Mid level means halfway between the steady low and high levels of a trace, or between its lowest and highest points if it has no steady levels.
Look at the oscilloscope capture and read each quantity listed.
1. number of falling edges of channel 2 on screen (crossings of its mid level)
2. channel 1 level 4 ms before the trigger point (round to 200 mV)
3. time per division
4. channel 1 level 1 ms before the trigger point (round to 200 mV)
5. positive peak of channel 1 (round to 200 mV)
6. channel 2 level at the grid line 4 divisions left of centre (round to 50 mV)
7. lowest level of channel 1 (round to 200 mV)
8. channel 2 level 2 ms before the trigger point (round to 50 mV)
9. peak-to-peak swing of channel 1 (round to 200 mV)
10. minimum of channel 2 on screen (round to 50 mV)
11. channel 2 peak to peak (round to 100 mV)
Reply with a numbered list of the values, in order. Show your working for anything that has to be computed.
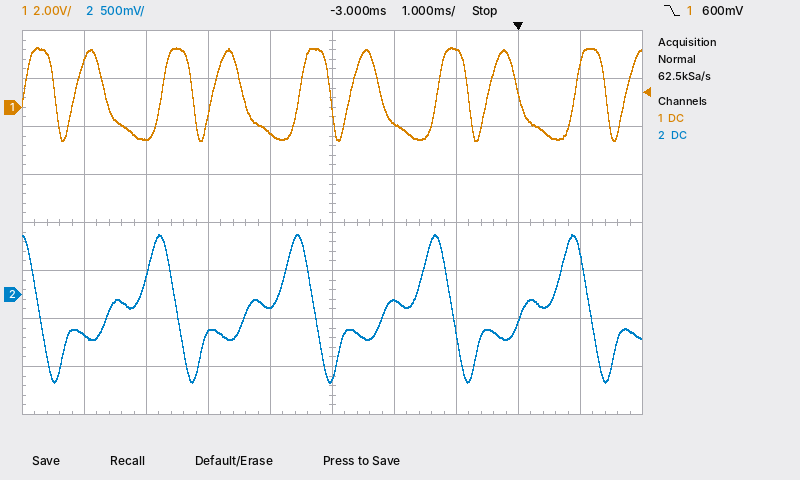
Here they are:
1. 5
2. -1.0 V
3. 1 ms
4. 2.4 V
5. 2.4 V
6. -400 mV
7. -1.4 V
8. -50 mV
9. 2.4 V − (-1.4 V) = 3.8 V
10. -900 mV
11. 1.50 V
